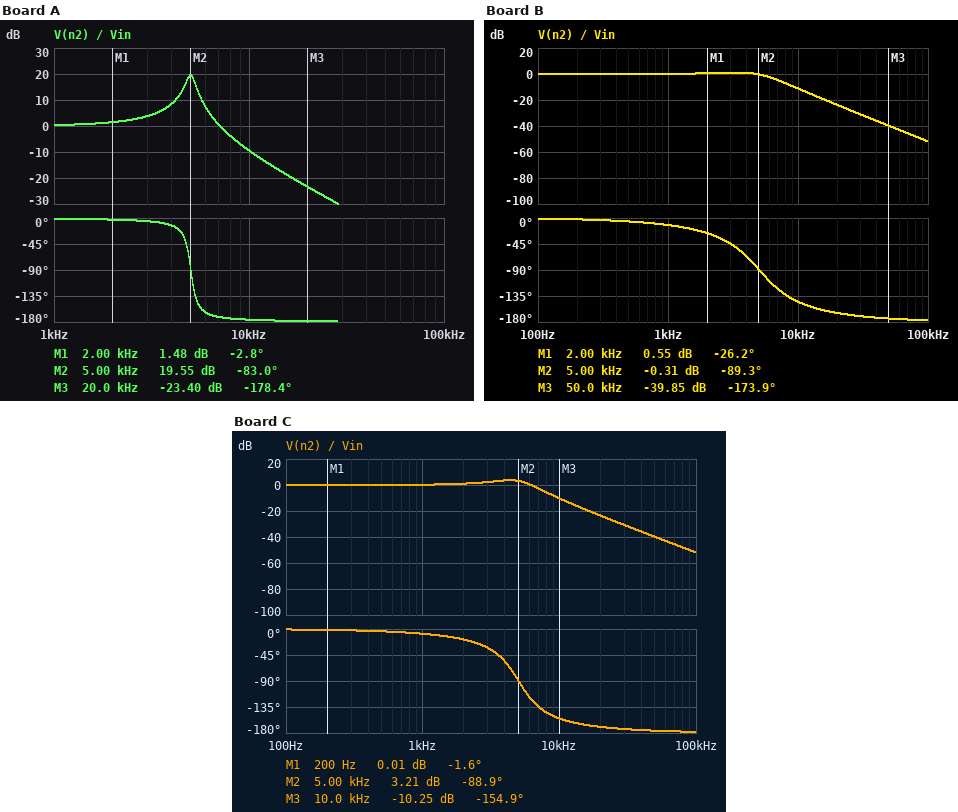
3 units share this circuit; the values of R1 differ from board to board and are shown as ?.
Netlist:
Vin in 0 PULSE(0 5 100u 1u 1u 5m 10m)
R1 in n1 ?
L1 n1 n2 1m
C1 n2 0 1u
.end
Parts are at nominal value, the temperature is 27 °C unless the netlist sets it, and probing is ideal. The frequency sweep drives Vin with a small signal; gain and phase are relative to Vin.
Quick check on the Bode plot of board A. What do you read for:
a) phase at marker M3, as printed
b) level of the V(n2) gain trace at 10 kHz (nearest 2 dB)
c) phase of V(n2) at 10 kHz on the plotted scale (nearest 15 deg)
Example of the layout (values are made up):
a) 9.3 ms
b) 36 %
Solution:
a) -178.4 deg
b) -10 dB
c) -180 deg
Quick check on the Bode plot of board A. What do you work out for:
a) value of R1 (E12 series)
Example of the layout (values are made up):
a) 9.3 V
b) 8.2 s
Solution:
a) 3.3 Ω
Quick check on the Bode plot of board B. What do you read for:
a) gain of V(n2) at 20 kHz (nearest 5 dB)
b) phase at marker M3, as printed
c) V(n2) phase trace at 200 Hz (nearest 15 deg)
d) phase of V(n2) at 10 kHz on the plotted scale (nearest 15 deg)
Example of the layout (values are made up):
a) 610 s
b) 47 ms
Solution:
a) -25 dB
b) -173.9 deg
c) 0 deg
d) -150 deg
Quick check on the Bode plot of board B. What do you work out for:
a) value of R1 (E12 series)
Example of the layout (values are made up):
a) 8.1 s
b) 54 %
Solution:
a) 33 Ω
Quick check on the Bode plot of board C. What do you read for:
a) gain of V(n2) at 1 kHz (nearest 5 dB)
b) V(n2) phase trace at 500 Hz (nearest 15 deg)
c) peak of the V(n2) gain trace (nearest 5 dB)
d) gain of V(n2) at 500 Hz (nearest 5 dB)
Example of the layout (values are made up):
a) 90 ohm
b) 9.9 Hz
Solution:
a) 0 dB
b) 0 deg
c) 5 dB
d) 0 dB
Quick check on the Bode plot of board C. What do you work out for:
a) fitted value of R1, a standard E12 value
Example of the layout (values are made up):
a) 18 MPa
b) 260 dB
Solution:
a) 22 Ω
